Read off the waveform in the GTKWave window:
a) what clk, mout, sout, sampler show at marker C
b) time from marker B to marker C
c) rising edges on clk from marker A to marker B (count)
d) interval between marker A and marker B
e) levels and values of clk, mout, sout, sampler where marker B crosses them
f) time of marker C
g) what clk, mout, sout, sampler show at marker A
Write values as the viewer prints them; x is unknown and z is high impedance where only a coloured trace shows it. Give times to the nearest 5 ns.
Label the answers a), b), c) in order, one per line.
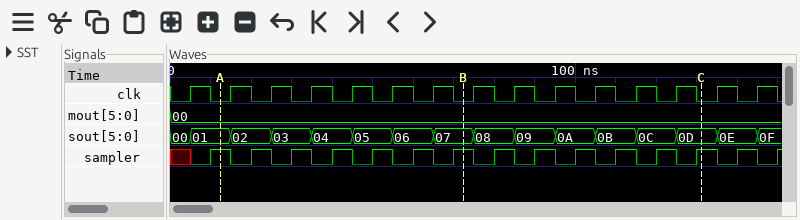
a) clk=0, mout=00, sout=0D, sampler=1
b) 60 ns
c) 6
d) 60 ns
e) clk=0, mout=00, sout=07, sampler=1
f) 130 ns
g) clk=0, mout=00, sout=01, sampler=1
